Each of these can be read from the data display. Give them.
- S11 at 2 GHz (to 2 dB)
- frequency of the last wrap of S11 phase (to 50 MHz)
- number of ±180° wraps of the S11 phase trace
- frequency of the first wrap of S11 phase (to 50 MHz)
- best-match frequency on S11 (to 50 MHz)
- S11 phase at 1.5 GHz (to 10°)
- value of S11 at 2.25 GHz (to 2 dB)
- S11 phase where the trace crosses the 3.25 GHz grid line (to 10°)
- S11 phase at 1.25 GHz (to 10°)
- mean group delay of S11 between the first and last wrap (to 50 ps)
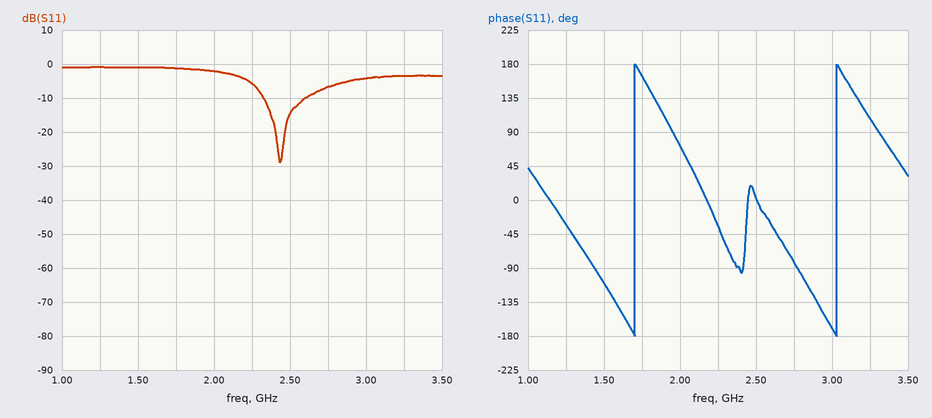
-2 dB
3.05 GHz
2
1.70 GHz
2.45 GHz
-110°
-6 dB
110°
-30°
750 ps
